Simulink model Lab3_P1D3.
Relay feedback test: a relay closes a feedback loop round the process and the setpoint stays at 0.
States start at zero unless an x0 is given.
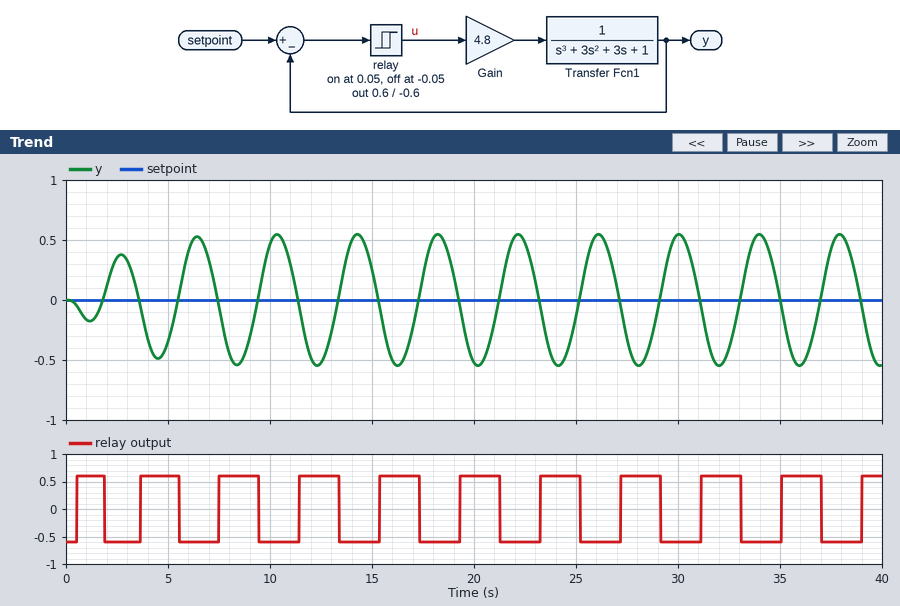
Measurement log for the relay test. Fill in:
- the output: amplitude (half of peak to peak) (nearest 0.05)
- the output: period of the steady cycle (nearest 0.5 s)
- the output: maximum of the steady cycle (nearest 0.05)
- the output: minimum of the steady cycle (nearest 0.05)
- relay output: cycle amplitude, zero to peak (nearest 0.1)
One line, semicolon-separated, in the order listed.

0.55; 4.0 s; 0.55; -0.55; 0.6
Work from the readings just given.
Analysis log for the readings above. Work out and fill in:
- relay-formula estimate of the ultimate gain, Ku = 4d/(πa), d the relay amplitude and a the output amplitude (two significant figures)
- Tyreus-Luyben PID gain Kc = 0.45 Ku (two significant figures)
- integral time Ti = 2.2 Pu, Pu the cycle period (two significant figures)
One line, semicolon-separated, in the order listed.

1.4; 0.63; 8.8 s
